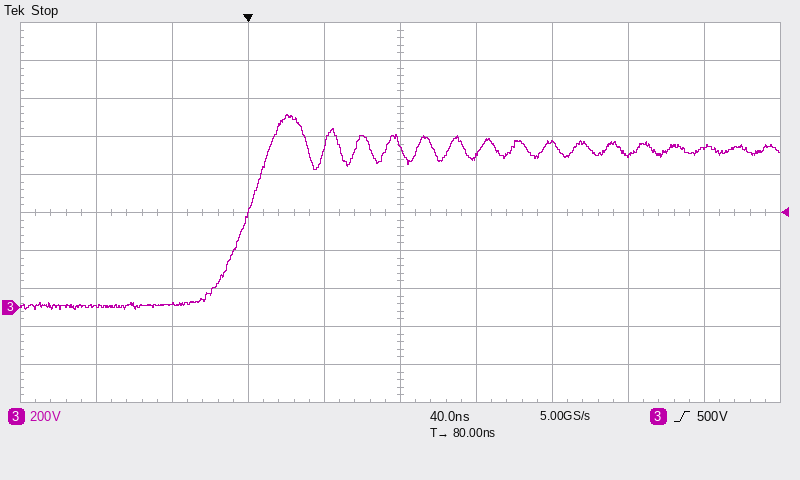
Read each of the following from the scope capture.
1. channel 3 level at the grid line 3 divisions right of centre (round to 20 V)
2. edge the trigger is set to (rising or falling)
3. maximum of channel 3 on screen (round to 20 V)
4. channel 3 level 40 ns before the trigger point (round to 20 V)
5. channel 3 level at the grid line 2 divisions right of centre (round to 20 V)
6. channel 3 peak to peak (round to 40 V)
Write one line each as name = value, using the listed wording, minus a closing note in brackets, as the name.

channel 3 level at the grid line 3 divisions right of centre = 800 V
edge the trigger is set to = rising
maximum of channel 3 on screen = 1.02 kV
channel 3 level 40 ns before the trigger point = 20 V
channel 3 level at the grid line 2 divisions right of centre = 860 V
channel 3 peak to peak = 1.04 kV
